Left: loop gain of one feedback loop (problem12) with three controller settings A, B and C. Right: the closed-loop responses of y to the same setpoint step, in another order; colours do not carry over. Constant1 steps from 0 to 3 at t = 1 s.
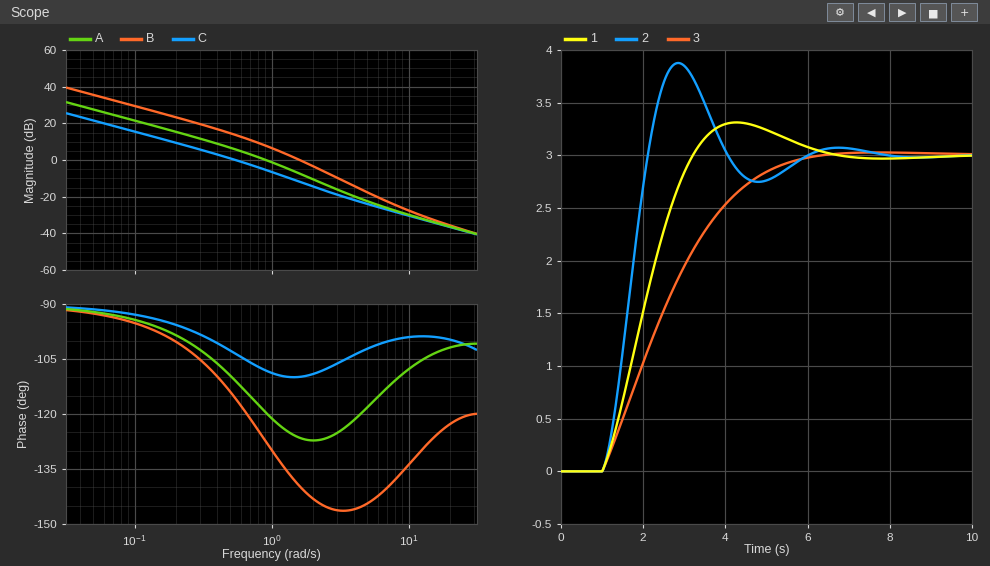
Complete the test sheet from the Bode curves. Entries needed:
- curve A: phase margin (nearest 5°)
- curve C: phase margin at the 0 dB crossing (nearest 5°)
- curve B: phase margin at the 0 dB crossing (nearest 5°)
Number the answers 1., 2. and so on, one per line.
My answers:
1. 60°
2. 75°
3. 40°
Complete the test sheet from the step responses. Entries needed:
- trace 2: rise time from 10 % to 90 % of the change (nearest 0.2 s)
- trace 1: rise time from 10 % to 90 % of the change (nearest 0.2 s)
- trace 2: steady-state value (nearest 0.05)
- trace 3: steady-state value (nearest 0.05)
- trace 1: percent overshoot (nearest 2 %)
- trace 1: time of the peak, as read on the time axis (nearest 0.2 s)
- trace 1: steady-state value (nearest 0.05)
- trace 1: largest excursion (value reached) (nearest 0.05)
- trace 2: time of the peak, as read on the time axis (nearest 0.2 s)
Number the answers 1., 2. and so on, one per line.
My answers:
1. 0.8 s
2. 1.6 s
3. 3.00
4. 3.00
5. 10 %
6. 4.2 s
7. 3.00
8. 3.30
9. 2.8 s
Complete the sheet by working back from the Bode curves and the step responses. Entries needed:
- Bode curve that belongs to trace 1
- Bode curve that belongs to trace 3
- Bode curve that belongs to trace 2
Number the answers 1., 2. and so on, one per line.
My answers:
1. A
2. C
3. B
